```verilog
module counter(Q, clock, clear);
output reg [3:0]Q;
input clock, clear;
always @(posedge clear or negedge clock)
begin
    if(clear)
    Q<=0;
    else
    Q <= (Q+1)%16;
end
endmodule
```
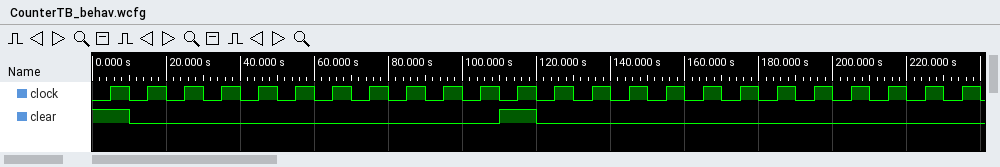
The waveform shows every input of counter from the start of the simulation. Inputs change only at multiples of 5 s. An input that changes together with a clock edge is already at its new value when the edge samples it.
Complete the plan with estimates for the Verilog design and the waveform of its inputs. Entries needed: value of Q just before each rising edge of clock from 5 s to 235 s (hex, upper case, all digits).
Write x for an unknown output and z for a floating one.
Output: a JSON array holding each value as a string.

["0, 1, 2, 3, 4, 5, 6, 7, 8, 9, A, 0, 1, 2, 3, 4, 5, 6, 7, 8, 9, A, B, C"]
